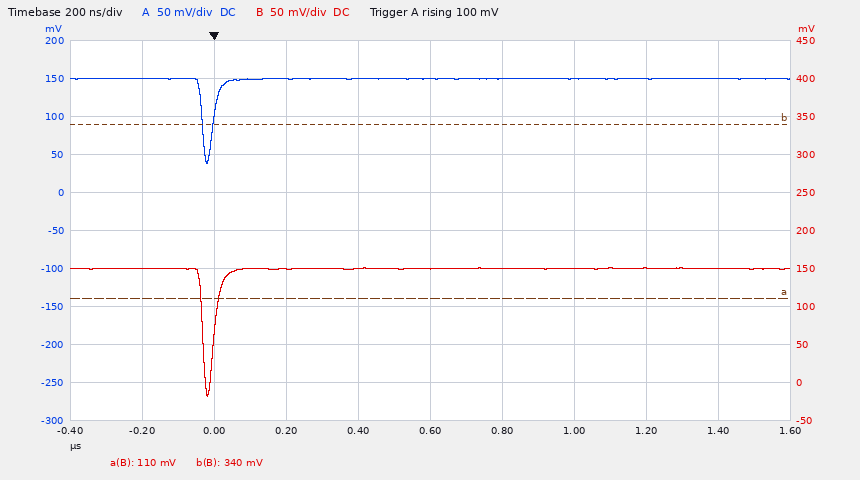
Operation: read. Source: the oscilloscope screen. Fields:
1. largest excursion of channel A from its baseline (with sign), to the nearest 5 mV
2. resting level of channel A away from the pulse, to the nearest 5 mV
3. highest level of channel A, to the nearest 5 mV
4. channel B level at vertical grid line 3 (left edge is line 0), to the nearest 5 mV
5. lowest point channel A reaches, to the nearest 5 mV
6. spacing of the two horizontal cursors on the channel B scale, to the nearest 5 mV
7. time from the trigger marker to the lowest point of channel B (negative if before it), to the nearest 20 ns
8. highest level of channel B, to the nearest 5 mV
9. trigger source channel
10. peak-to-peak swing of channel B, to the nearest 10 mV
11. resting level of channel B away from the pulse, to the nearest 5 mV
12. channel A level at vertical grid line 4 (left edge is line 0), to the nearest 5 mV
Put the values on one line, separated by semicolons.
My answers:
-110 mV; 150 mV; 150 mV; 150 mV; 40 mV; 230 mV; -20 ns; 150 mV; channel A; 170 mV; 150 mV; 150 mV
